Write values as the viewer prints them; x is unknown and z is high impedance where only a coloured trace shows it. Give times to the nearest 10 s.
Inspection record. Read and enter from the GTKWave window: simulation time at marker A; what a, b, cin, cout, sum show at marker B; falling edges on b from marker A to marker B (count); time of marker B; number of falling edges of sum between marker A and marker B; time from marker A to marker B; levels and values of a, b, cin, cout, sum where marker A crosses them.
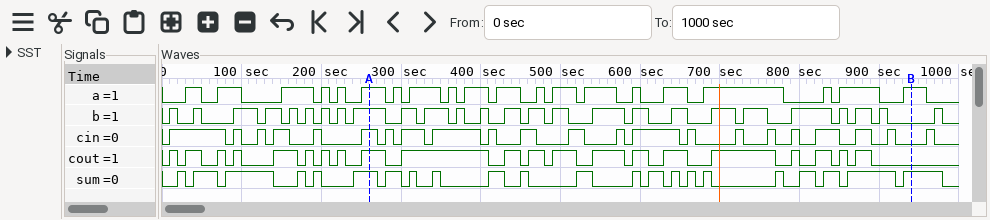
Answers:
260 s
a=1, b=0, cin=0, cout=0, sum=1
17
940 s
16
680 s
a=1, b=1, cin=1, cout=1, sum=1
